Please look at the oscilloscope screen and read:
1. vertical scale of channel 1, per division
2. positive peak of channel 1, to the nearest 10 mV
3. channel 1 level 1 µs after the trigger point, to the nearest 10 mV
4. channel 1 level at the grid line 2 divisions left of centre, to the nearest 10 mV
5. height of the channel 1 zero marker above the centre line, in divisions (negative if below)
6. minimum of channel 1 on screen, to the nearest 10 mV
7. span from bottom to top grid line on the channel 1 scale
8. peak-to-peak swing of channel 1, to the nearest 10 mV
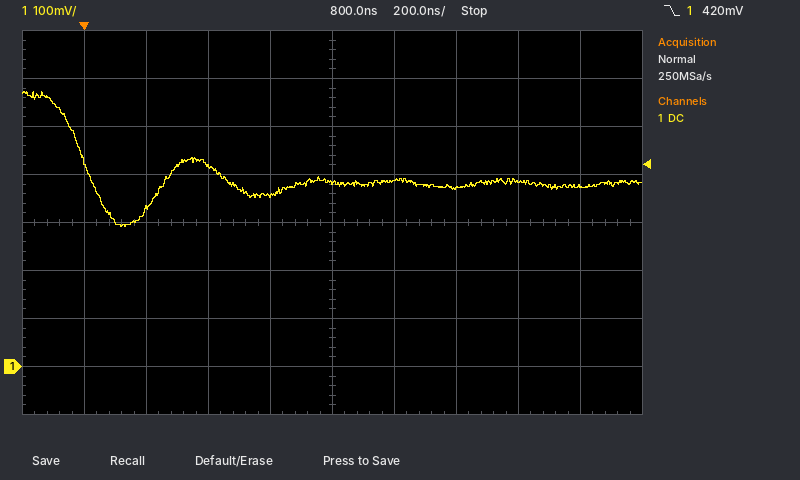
100 mV
570 mV
390 mV
420 mV
-3.0 div
290 mV
800 mV
280 mV
